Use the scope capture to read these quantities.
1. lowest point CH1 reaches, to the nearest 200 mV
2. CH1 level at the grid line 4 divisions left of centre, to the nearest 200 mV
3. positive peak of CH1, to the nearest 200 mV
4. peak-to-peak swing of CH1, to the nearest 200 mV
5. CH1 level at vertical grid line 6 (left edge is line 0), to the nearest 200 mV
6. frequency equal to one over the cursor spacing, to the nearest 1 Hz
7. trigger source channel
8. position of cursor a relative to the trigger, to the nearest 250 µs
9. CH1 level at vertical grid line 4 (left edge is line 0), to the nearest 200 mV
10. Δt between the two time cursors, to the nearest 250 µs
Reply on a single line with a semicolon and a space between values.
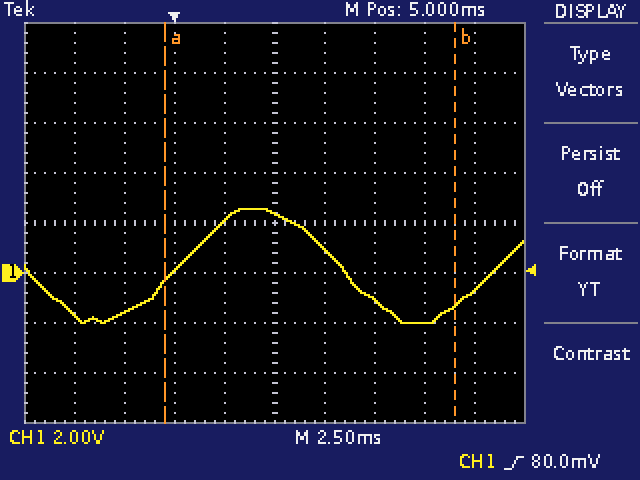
-2.0 V; -1.6 V; 2.6 V; 4.6 V; 1.0 V; 69 Hz; CH1; -500 µs; 2.0 V; 14.50 ms
